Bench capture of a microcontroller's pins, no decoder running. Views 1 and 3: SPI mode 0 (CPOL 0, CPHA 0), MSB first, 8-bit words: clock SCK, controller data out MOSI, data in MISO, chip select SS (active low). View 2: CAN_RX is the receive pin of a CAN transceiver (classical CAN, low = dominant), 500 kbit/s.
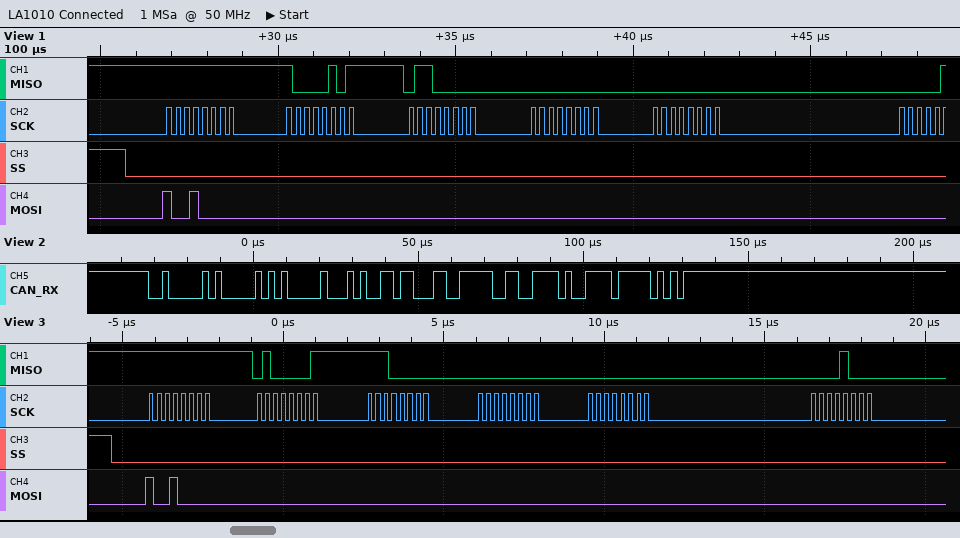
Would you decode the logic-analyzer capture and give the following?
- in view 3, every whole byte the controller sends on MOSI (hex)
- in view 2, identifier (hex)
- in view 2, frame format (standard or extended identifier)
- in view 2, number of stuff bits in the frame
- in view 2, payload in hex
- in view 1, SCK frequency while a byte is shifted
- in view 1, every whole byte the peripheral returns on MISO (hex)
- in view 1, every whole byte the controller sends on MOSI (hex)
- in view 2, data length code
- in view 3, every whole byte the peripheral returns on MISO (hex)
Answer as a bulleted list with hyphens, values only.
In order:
- 90 00 00 00 00 00
- 0x204
- standard
- 5
- 00 A6 C6 7D 9E
- 4 MHz
- FF 85 60 00 00
- 90 00 00 00 00
- 5
- FF 41 E0 00 00 08
